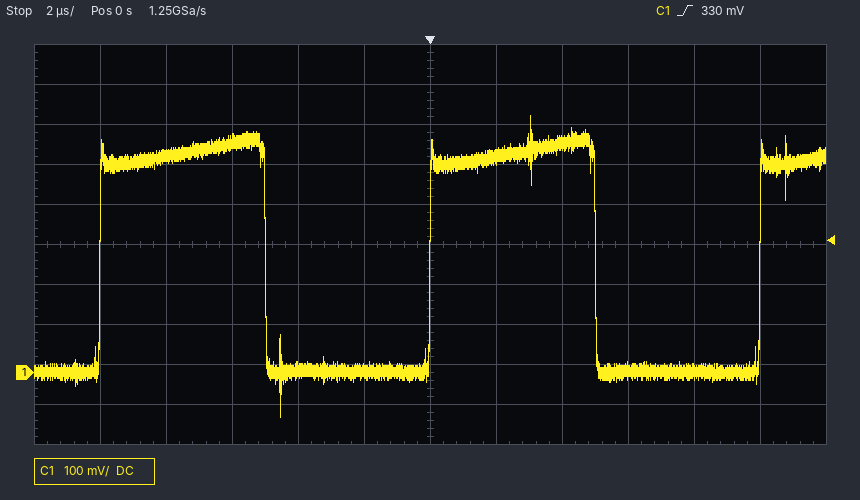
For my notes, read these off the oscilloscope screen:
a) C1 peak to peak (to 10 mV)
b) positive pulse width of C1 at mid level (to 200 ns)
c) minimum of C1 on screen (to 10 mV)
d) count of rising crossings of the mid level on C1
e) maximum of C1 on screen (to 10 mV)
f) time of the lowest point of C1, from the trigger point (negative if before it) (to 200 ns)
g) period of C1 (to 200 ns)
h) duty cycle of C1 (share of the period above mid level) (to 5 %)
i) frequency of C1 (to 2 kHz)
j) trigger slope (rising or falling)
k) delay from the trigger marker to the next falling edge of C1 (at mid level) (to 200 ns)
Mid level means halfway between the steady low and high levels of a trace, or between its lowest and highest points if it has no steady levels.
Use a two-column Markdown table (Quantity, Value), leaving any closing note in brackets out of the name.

| Quantity | Value |
|---|---|
| C1 peak to peak | 750 mV |
| positive pulse width of C1 at mid level | 5.0 µs |
| minimum of C1 on screen | -110 mV |
| count of rising crossings of the mid level on C1 | 3 |
| maximum of C1 on screen | 640 mV |
| time of the lowest point of C1, from the trigger point (negative if before it) | -4.6 µs |
| period of C1 | 10.0 µs |
| duty cycle of C1 (share of the period above mid level) | 50 % |
| frequency of C1 | 100 kHz |
| trigger slope | rising |
| delay from the trigger marker to the next falling edge of C1 (at mid level) | 5.0 µs |
